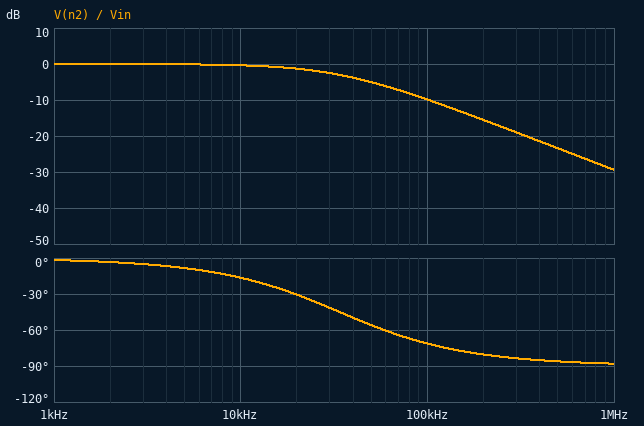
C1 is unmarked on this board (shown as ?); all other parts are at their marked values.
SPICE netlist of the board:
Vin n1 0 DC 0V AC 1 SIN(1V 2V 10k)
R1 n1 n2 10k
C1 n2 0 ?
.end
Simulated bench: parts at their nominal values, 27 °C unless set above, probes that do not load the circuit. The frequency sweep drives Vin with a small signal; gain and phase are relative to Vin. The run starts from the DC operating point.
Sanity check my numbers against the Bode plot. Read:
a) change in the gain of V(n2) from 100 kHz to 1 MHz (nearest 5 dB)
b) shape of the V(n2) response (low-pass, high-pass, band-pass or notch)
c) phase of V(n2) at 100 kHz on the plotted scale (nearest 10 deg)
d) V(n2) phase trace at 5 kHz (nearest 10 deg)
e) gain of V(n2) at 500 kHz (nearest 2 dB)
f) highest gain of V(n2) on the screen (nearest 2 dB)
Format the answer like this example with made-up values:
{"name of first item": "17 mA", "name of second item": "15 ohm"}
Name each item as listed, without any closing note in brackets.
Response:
{"change in the gain of V(n2) from 100 kHz to 1 MHz": "-20 dB", "shape of the V(n2) response": "low-pass", "phase of V(n2) at 100 kHz on the plotted scale": "-70 deg", "V(n2) phase trace at 5 kHz": "-10 deg", "gain of V(n2) at 500 kHz": "-24 dB", "highest gain of V(n2) on the screen": "0 dB"}
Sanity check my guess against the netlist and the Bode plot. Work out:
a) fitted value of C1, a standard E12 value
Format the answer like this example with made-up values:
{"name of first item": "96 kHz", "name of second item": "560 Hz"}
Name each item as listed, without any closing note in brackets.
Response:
{"fitted value of C1, a standard E12 value": "470 pF"}
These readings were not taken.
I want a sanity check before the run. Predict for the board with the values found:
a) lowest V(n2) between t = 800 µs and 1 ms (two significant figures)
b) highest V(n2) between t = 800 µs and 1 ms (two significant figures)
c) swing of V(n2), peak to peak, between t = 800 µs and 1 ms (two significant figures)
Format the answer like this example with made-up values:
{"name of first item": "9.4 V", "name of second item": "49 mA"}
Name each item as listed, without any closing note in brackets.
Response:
{"lowest V(n2) between t = 800 µs and 1 ms": "-920 mV", "highest V(n2) between t = 800 µs and 1 ms": "2.9 V", "swing of V(n2), peak to peak, between t = 800 µs and 1 ms": "3.8 V"}
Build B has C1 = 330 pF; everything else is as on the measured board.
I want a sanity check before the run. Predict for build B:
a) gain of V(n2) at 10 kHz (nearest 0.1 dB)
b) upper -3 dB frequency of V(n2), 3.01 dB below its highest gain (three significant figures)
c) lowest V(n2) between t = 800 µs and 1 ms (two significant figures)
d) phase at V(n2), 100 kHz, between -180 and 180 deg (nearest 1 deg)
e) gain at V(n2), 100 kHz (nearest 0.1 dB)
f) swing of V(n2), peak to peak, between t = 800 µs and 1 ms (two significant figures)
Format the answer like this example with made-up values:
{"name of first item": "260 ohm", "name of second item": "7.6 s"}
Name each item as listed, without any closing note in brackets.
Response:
{"gain of V(n2) at 10 kHz": "-0.2 dB", "upper -3 dB frequency of V(n2), 3.01 dB below its highest gain": "48.2 kHz", "lowest V(n2) between t = 800 µs and 1 ms": "-960 mV", "phase at V(n2), 100 kHz, between -180 and 180 deg": "-64 deg", "gain at V(n2), 100 kHz": "-7.2 dB", "swing of V(n2), peak to peak, between t = 800 µs and 1 ms": "3.9 V"}
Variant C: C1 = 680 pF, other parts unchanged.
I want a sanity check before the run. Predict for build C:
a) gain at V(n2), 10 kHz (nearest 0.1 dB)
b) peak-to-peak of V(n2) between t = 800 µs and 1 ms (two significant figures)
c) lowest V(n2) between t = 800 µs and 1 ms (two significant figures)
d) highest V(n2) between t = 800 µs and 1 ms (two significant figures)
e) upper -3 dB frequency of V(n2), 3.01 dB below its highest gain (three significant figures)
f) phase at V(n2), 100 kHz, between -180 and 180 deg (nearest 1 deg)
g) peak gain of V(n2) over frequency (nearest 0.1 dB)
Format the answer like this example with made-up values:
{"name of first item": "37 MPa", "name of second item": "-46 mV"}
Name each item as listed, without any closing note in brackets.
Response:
{"gain at V(n2), 10 kHz": "-0.7 dB", "peak-to-peak of V(n2) between t = 800 µs and 1 ms": "3.7 V", "lowest V(n2) between t = 800 µs and 1 ms": "-840 mV", "highest V(n2) between t = 800 µs and 1 ms": "2.8 V", "upper -3 dB frequency of V(n2), 3.01 dB below its highest gain": "23.4 kHz", "phase at V(n2), 100 kHz, between -180 and 180 deg": "-77 deg", "peak gain of V(n2) over frequency": "0 dB"}
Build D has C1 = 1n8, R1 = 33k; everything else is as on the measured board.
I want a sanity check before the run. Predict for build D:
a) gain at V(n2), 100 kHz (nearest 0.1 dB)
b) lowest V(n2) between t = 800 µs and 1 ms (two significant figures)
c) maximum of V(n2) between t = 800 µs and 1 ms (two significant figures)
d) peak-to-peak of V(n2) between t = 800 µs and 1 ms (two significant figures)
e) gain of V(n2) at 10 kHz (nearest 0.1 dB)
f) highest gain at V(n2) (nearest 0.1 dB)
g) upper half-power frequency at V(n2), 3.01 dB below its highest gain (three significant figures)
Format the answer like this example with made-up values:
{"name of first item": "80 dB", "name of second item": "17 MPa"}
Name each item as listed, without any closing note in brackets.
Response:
{"gain at V(n2), 100 kHz": "-31.4 dB", "lowest V(n2) between t = 800 µs and 1 ms": "480 mV", "maximum of V(n2) between t = 800 µs and 1 ms": "1.5 V", "peak-to-peak of V(n2) between t = 800 µs and 1 ms": "1.0 V", "gain of V(n2) at 10 kHz": "-11.7 dB", "highest gain at V(n2)": "0 dB", "upper half-power frequency at V(n2), 3.01 dB below its highest gain": "2.68 kHz"}
